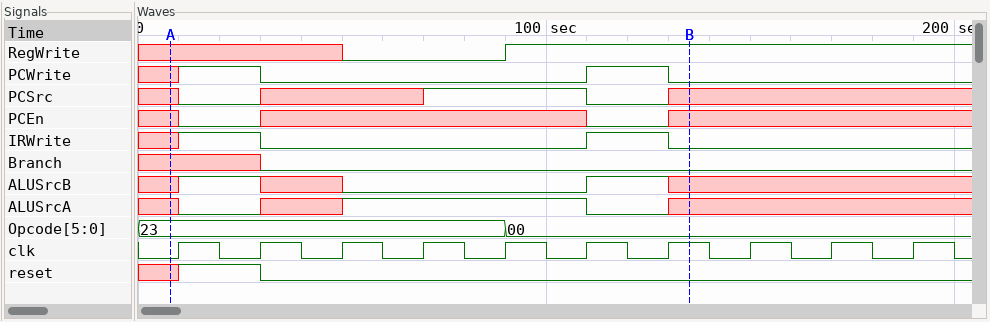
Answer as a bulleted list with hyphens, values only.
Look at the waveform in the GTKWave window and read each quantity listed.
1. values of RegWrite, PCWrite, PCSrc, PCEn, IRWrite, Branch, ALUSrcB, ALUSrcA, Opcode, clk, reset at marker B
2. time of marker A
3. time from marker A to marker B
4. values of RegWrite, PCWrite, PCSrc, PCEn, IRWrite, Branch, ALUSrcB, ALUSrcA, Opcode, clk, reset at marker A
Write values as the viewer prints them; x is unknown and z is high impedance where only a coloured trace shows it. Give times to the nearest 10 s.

- RegWrite=1, PCWrite=0, PCSrc=x, PCEn=x, IRWrite=0, Branch=0, ALUSrcB=x, ALUSrcA=x, Opcode=00, clk=1, reset=0
- 10 s
- 130 s
- RegWrite=x, PCWrite=x, PCSrc=x, PCEn=x, IRWrite=x, Branch=x, ALUSrcB=x, ALUSrcA=x, Opcode=23, clk=0, reset=x
